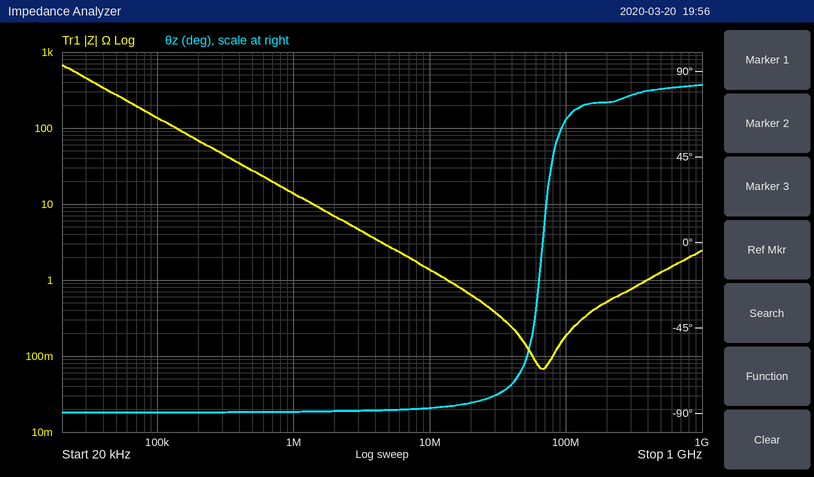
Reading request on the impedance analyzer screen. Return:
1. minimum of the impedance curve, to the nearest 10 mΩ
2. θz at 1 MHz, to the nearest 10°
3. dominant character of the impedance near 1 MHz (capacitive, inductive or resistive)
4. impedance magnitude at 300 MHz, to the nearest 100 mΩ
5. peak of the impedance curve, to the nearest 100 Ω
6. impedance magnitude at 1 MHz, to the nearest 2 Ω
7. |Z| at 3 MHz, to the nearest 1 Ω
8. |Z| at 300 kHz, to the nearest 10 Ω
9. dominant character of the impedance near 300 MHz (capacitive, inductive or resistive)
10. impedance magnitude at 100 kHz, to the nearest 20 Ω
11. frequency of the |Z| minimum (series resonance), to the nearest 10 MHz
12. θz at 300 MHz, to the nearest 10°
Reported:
70 mΩ
-90°
capacitive
800 mΩ
700 Ω
14 Ω
5 Ω
50 Ω
inductive
140 Ω
70 MHz
80°
